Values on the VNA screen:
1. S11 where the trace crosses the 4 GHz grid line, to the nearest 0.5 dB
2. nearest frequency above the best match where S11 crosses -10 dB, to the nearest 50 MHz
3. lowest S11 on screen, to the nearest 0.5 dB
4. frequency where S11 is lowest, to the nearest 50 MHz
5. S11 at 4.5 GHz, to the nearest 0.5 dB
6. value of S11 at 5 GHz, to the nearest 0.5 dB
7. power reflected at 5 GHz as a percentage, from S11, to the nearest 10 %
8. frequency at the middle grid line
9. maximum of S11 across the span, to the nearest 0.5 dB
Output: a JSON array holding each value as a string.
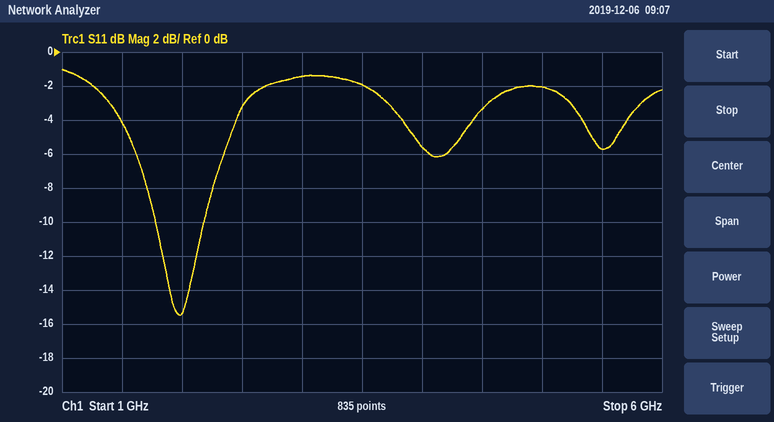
["-5.5 dB", "2.20 GHz", "-15.5 dB", "2.00 GHz", "-3.5 dB", "-2.0 dB", "60 %", "3.5 GHz", "-1.0 dB"]
